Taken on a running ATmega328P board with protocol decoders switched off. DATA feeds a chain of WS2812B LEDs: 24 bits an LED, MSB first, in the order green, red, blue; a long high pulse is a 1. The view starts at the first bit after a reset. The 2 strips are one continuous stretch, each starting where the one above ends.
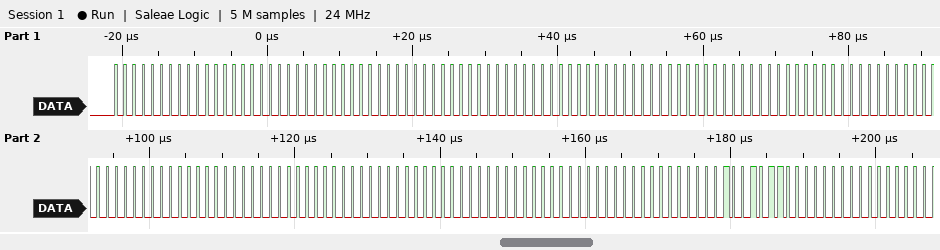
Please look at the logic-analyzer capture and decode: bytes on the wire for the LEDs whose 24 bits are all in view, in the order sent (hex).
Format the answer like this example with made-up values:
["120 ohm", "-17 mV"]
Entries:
["00 00 00 00 00 00 00 00 00 00 00 00 00 00 00 00 00 00 00 00 96"]
